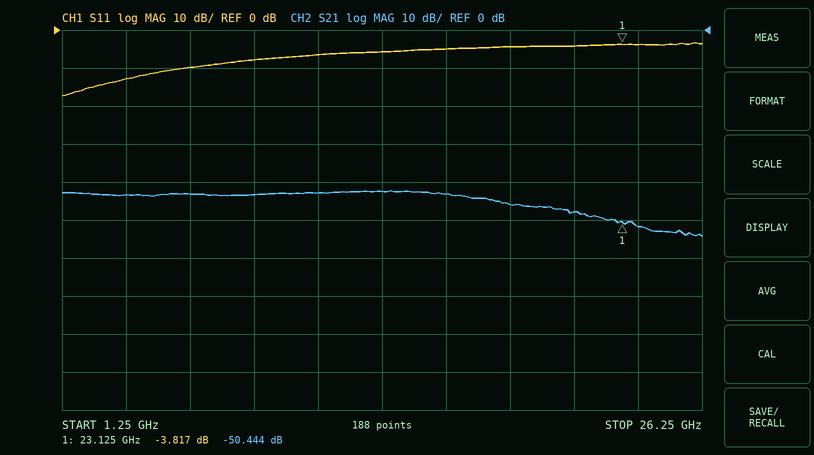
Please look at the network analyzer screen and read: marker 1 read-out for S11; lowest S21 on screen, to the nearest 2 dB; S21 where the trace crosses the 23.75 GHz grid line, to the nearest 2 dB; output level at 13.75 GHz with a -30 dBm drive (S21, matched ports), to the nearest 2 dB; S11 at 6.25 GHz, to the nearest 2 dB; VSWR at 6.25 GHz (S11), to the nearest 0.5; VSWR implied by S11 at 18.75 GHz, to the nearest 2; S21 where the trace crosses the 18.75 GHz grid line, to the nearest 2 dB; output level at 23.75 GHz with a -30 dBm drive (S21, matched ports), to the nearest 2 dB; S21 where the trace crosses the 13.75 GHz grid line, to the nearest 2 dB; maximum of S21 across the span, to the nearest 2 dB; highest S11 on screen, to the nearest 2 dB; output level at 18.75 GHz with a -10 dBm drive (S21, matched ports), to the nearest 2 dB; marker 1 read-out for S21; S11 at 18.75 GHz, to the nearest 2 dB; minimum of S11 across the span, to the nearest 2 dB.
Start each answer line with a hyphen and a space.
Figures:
- -3.817 dB
- -54 dB
- -52 dB
- -72 dBm
- -10 dB
- 2.0
- 4
- -46 dB
- -82 dBm
- -42 dB
- -42 dB
- -4 dB
- -56 dBm
- -50.444 dB
- -4 dB
- -18 dB
